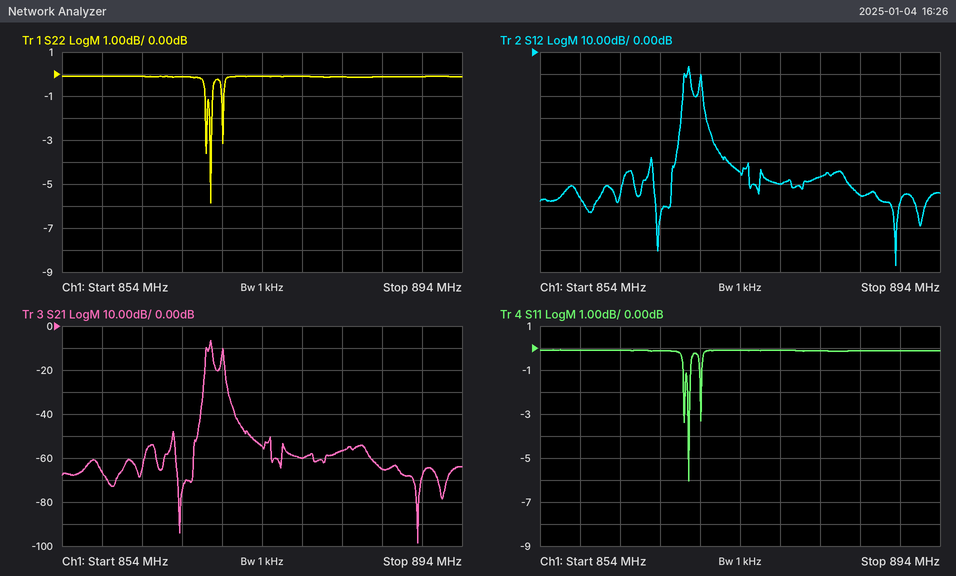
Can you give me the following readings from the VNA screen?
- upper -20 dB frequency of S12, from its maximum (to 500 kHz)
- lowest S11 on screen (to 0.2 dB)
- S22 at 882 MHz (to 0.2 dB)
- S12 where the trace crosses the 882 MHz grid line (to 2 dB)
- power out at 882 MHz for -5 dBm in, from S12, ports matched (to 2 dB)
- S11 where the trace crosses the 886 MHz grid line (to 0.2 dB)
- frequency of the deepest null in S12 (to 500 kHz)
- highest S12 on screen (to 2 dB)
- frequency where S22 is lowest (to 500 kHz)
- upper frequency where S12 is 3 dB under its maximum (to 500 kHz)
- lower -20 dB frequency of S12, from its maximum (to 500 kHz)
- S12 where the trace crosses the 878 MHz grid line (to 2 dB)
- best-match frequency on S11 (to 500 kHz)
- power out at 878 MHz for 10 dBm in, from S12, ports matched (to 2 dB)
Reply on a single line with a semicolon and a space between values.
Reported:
870.5 MHz; -6.0 dB; -0.2 dB; -56 dB; -62 dBm; -0.2 dB; 889.5 MHz; -6 dB; 869.0 MHz; 869.0 MHz; 868.0 MHz; -60 dB; 869.0 MHz; -50 dBm
